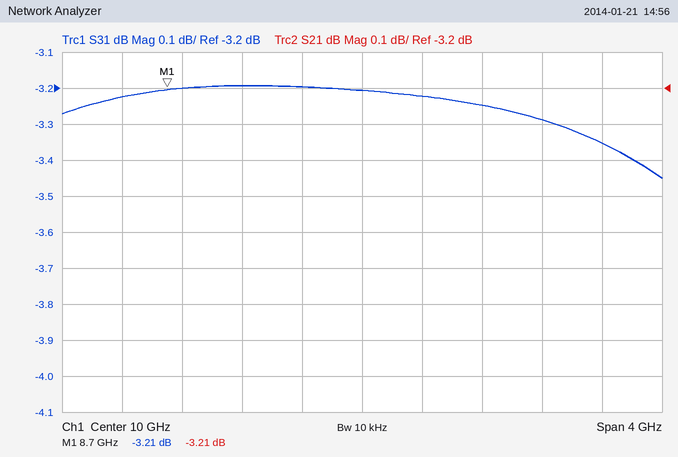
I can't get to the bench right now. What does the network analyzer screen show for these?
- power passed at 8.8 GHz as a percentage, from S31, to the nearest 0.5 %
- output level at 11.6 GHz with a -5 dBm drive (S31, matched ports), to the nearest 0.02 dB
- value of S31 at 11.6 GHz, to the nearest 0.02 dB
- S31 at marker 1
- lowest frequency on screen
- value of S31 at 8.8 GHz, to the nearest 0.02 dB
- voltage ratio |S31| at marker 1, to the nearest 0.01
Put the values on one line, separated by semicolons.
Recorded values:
48.0 %; -8.36 dBm; -3.36 dB; -3.21 dB; 8 GHz; -3.20 dB; 0.69
